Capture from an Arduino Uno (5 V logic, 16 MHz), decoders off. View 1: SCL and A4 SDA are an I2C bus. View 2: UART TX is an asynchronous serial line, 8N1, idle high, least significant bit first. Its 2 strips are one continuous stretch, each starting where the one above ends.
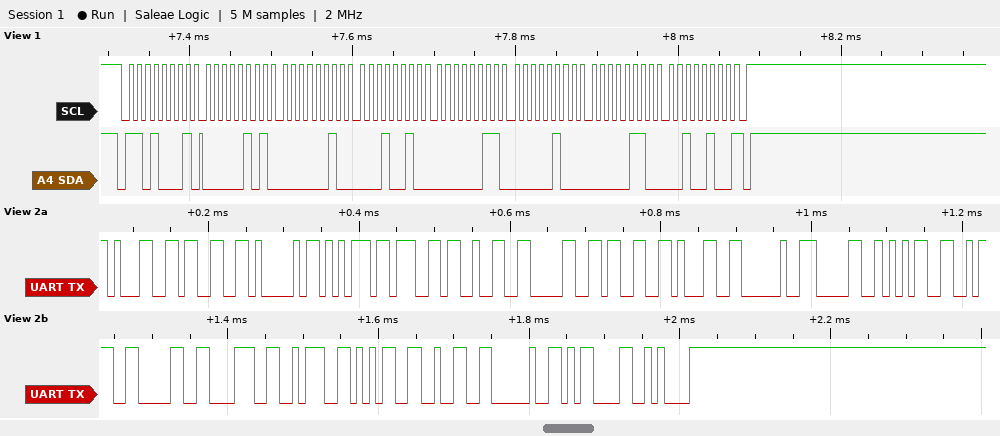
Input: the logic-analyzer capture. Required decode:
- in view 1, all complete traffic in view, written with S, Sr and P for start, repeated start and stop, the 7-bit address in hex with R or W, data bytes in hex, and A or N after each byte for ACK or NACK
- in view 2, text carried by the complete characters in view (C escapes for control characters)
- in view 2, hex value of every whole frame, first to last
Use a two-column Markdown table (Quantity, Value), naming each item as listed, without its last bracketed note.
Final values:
| Quantity | Value |
|---|---|
| in view 1, all complete traffic in view, written with S, Sr and P for start, repeated start and stop, the 7-bit address in hex with R or W, data bytes in hex, and A or N after each byte for ACK or NACK | S 68R A 05 A 02 A 12 A 03 A 04 A 06 A 24 N P |
| in view 2, text carried by the complete characters in view | "13Aug2031 05:08:52 \r\n" |
| in view 2, hex value of every whole frame, first to last | 31 33 41 75 67 32 30 33 31 20 30 35 3A 30 38 3A 35 32 20 0D 0A |
